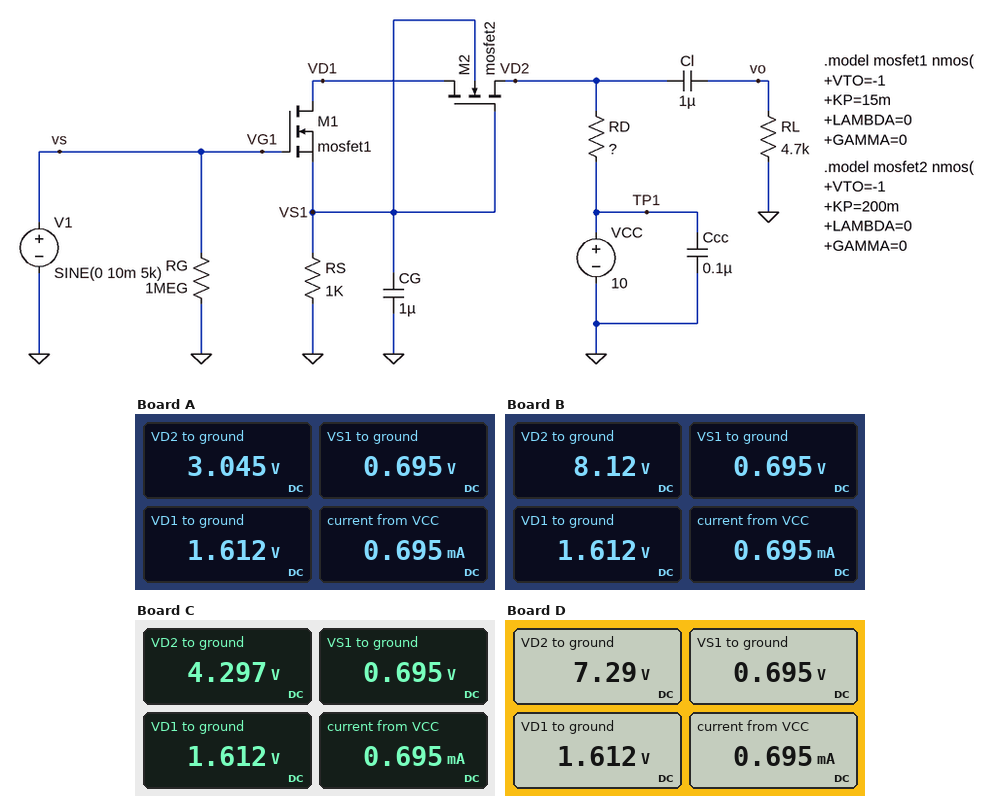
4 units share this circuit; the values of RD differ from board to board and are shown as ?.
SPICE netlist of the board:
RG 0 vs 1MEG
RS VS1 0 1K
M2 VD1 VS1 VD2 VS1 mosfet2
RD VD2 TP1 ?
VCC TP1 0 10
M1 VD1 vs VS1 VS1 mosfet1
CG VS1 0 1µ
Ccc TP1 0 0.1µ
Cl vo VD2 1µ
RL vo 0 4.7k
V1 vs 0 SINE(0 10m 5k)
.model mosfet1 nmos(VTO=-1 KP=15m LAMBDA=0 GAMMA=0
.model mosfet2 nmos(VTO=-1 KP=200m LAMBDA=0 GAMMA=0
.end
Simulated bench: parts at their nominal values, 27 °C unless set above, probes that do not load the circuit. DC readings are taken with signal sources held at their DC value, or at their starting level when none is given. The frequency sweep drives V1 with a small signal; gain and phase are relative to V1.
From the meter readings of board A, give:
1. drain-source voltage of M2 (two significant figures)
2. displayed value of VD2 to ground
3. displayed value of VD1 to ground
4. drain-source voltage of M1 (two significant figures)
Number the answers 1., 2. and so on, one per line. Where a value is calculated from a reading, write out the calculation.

1. 1.612 V - 3.045 V = -1.4 V
2. 3.045 V
3. 1.612 V
4. 1.612 V - 695 mV = 920 mV
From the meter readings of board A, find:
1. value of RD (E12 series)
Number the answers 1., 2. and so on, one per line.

1. 10 kΩ
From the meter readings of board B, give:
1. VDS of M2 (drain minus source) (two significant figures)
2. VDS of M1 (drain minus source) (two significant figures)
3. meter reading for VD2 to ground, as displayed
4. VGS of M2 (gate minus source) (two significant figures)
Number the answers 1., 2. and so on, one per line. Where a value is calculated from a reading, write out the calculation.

1. 1.612 V - 8.12 V = -6.5 V
2. 1.612 V - 695 mV = 920 mV
3. 8.12 V
4. 695 mV - 8.12 V = -7.4 V
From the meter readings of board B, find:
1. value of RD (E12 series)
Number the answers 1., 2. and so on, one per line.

1. 2.7 kΩ
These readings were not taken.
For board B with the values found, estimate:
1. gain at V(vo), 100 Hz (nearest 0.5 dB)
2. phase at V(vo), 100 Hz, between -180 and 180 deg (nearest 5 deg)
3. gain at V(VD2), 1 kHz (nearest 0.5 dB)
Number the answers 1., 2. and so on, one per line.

1. 4.0 dB
2. -140 deg
3. 15.5 dB
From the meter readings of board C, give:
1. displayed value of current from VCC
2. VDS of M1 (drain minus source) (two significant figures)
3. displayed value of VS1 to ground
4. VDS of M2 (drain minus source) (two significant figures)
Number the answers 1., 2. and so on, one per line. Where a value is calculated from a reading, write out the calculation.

1. 0.695 mA
2. 1.612 V - 695 mV = 920 mV
3. 0.695 V
4. 1.612 V - 4.297 V = -2.7 V
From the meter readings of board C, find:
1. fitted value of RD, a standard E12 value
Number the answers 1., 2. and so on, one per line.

1. 8.2 kΩ
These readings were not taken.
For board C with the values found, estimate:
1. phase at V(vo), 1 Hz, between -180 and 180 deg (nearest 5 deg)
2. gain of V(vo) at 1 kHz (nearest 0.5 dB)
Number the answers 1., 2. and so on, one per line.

1. -95 deg
2. 20.5 dB
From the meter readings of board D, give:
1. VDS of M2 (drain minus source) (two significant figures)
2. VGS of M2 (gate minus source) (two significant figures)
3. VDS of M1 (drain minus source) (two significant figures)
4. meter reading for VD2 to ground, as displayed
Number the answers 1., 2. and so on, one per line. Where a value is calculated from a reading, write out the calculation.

1. 1.612 V - 7.29 V = -5.7 V
2. 695 mV - 7.29 V = -6.6 V
3. 1.612 V - 695 mV = 920 mV
4. 7.29 V
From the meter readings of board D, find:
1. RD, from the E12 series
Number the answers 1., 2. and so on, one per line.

1. 3.9 kΩ
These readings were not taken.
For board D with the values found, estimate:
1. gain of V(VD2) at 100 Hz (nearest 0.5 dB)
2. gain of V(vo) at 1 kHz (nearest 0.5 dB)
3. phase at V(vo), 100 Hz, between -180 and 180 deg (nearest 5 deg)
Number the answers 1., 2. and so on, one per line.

1. 6.5 dB
2. 17.5 dB
3. -145 deg
